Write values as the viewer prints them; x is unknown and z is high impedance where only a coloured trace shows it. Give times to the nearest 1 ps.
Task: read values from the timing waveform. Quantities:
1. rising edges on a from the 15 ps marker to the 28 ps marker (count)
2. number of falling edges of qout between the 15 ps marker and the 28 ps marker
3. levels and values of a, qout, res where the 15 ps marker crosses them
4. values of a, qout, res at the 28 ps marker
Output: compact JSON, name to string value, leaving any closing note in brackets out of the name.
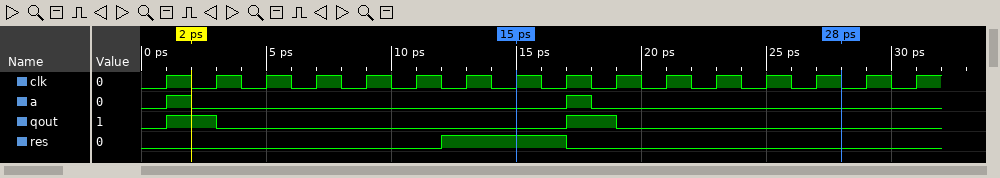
{"rising edges on a from the 15 ps marker to the 28 ps marker": "1", "number of falling edges of qout between the 15 ps marker and the 28 ps marker": "1", "levels and values of a, qout, res where the 15 ps marker crosses them": "a=0, qout=0, res=1", "values of a, qout, res at the 28 ps marker": "a=0, qout=0, res=0"}
